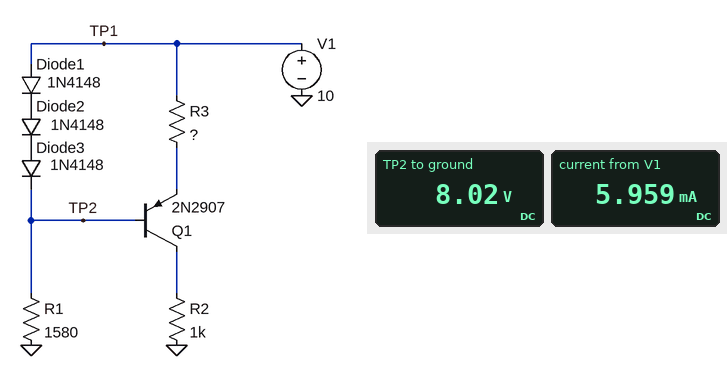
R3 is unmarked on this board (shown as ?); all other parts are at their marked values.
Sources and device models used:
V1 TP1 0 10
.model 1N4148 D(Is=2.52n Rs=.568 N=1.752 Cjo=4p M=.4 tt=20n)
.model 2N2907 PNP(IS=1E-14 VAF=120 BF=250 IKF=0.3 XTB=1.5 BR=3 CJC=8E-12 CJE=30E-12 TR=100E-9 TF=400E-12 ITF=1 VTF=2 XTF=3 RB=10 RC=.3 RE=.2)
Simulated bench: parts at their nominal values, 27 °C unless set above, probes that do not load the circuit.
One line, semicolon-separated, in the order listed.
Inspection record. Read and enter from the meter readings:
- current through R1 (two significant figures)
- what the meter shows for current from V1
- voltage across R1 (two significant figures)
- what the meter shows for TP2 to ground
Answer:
5.1 mA; 5.959 mA; 8.0 V; 8.02 V
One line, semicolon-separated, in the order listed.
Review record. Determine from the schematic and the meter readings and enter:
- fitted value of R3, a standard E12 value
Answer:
1.5 kΩ
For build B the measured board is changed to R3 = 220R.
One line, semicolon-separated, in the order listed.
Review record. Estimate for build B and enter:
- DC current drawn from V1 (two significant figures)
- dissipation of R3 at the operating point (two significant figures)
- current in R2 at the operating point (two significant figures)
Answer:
11 mA; 7.4 mW; 5.8 mA
